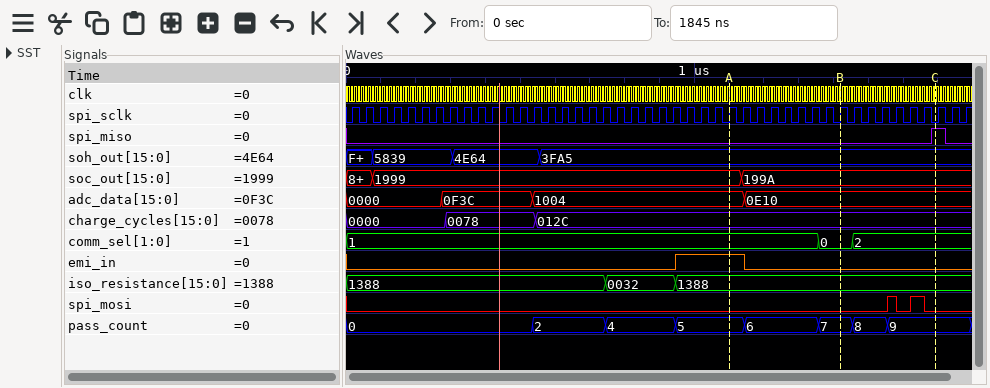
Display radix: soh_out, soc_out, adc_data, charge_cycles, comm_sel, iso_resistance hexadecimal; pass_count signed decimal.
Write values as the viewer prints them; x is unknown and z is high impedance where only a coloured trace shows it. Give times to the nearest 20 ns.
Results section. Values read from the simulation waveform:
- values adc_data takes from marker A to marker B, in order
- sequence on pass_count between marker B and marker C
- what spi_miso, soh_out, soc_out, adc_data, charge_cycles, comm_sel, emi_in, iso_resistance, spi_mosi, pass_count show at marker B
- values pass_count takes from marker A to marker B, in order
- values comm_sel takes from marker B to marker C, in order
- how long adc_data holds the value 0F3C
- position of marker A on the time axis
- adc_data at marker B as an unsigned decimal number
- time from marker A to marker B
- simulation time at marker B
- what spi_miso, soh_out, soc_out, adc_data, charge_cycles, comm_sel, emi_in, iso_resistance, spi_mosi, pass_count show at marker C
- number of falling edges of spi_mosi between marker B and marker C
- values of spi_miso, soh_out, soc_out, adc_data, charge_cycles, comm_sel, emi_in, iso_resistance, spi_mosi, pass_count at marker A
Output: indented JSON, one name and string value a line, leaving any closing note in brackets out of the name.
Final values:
{
  "values adc_data takes from marker A to marker B, in order": "1004, 0E10",
  "sequence on pass_count between marker B and marker C": "7, 8, 9",
  "what spi_miso, soh_out, soc_out, adc_data, charge_cycles, comm_sel, emi_in, iso_resistance, spi_mosi, pass_count show at marker B": "spi_miso=0, soh_out=3FA5, soc_out=199A, adc_data=0E10, charge_cycles=012C, comm_sel=0, emi_in=0, iso_resistance=1388, spi_mosi=0, pass_count=7",
  "values pass_count takes from marker A to marker B, in order": "5, 6, 7",
  "values comm_sel takes from marker B to marker C, in order": "0, 2",
  "how long adc_data holds the value 0F3C": "260 ns",
  "position of marker A on the time axis": "1100 ns",
  "adc_data at marker B as an unsigned decimal number": "3600",
  "time from marker A to marker B": "320 ns",
  "simulation time at marker B": "1420 ns",
  "what spi_miso, soh_out, soc_out, adc_data, charge_cycles, comm_sel, emi_in, iso_resistance, spi_mosi, pass_count show at marker C": "spi_miso=1, soh_out=3FA5, soc_out=199A, adc_data=0E10, charge_cycles=012C, comm_sel=2, emi_in=0, iso_resistance=1388, spi_mosi=0, pass_count=9",
  "number of falling edges of spi_mosi between marker B and marker C": "2",
  "values of spi_miso, soh_out, soc_out, adc_data, charge_cycles, comm_sel, emi_in, iso_resistance, spi_mosi, pass_count at marker A": "spi_miso=0, soh_out=3FA5, soc_out=1999, adc_data=1004, charge_cycles=012C, comm_sel=1, emi_in=1, iso_resistance=1388, spi_mosi=0, pass_count=5"
}
